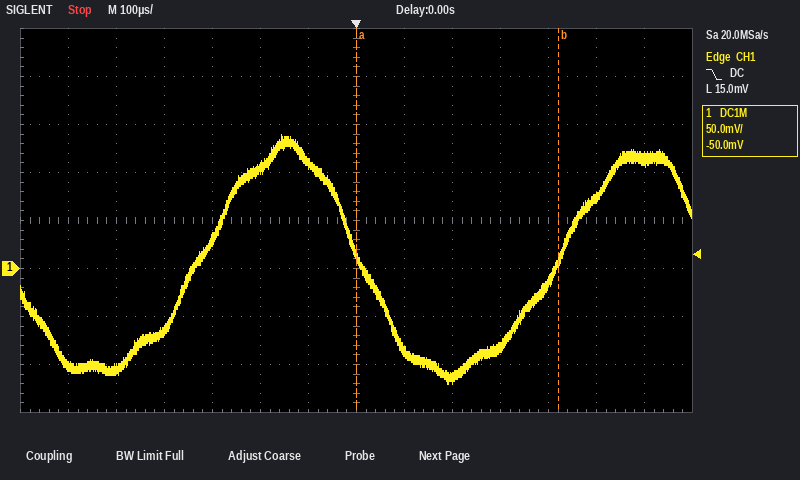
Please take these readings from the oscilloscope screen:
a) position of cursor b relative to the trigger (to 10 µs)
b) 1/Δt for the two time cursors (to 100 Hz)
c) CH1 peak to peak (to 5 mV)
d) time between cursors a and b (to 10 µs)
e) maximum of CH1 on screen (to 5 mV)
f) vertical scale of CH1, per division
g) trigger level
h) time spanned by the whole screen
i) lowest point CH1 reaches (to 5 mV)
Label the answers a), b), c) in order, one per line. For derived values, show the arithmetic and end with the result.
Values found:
a) +420 µs
b) 1 / 420 µs ≈ 2.4 kHz
c) 140 mV − (-120 mV) = 260 mV
d) 420 µs
e) 140 mV
f) 50 mV
g) 15.0 mV
h) 1.4 ms
i) -120 mV
